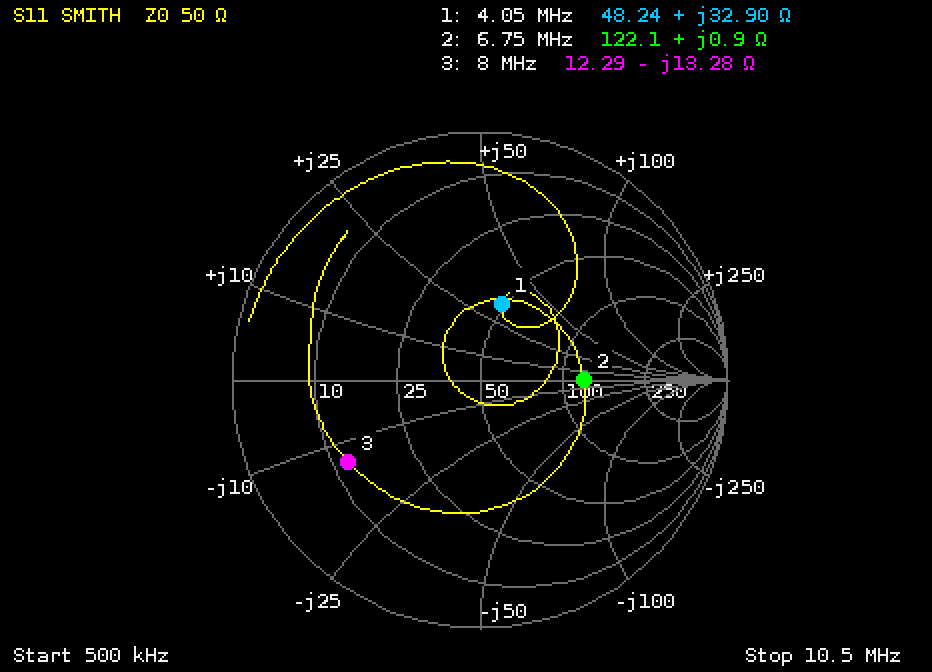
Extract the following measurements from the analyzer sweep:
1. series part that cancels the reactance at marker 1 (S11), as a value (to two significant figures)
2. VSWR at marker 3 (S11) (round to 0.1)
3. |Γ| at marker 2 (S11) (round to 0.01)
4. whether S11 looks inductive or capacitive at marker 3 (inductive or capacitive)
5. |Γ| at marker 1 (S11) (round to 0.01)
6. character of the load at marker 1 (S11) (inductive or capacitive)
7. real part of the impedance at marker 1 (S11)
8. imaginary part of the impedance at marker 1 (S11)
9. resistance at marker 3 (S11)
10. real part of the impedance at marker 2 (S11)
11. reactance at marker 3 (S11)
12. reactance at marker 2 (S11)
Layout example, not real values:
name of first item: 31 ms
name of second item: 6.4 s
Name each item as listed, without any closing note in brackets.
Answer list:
series part that cancels the reactance at marker 1 (S11), as a value: 1.2 nF
VSWR at marker 3 (S11): 4.4
|Γ| at marker 2 (S11): 0.42
whether S11 looks inductive or capacitive at marker 3: capacitive
|Γ| at marker 1 (S11): 0.32
character of the load at marker 1 (S11): inductive
real part of the impedance at marker 1: 48.24 Ω
imaginary part of the impedance at marker 1: +32.90 Ω
resistance at marker 3: 12.29 Ω
real part of the impedance at marker 2: 122.1 Ω
reactance at marker 3: -13.28 Ω
reactance at marker 2: +0.9 Ω
